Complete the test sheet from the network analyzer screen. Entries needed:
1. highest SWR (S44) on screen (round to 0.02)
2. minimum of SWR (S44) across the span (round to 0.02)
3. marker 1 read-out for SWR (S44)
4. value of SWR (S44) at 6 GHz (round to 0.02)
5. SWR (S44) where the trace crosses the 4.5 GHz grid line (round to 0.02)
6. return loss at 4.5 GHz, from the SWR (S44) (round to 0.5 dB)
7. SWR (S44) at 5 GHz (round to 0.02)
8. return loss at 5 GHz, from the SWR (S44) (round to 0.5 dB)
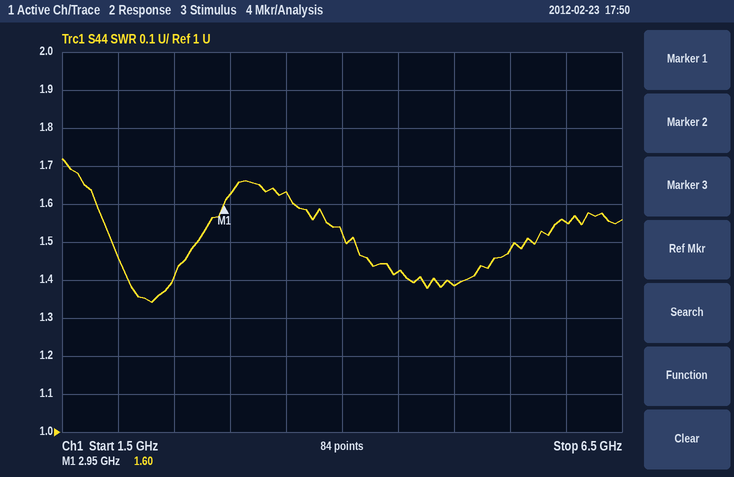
1.72
1.34
1.60
1.56
1.42
15.0 dB
1.38
16.0 dB
